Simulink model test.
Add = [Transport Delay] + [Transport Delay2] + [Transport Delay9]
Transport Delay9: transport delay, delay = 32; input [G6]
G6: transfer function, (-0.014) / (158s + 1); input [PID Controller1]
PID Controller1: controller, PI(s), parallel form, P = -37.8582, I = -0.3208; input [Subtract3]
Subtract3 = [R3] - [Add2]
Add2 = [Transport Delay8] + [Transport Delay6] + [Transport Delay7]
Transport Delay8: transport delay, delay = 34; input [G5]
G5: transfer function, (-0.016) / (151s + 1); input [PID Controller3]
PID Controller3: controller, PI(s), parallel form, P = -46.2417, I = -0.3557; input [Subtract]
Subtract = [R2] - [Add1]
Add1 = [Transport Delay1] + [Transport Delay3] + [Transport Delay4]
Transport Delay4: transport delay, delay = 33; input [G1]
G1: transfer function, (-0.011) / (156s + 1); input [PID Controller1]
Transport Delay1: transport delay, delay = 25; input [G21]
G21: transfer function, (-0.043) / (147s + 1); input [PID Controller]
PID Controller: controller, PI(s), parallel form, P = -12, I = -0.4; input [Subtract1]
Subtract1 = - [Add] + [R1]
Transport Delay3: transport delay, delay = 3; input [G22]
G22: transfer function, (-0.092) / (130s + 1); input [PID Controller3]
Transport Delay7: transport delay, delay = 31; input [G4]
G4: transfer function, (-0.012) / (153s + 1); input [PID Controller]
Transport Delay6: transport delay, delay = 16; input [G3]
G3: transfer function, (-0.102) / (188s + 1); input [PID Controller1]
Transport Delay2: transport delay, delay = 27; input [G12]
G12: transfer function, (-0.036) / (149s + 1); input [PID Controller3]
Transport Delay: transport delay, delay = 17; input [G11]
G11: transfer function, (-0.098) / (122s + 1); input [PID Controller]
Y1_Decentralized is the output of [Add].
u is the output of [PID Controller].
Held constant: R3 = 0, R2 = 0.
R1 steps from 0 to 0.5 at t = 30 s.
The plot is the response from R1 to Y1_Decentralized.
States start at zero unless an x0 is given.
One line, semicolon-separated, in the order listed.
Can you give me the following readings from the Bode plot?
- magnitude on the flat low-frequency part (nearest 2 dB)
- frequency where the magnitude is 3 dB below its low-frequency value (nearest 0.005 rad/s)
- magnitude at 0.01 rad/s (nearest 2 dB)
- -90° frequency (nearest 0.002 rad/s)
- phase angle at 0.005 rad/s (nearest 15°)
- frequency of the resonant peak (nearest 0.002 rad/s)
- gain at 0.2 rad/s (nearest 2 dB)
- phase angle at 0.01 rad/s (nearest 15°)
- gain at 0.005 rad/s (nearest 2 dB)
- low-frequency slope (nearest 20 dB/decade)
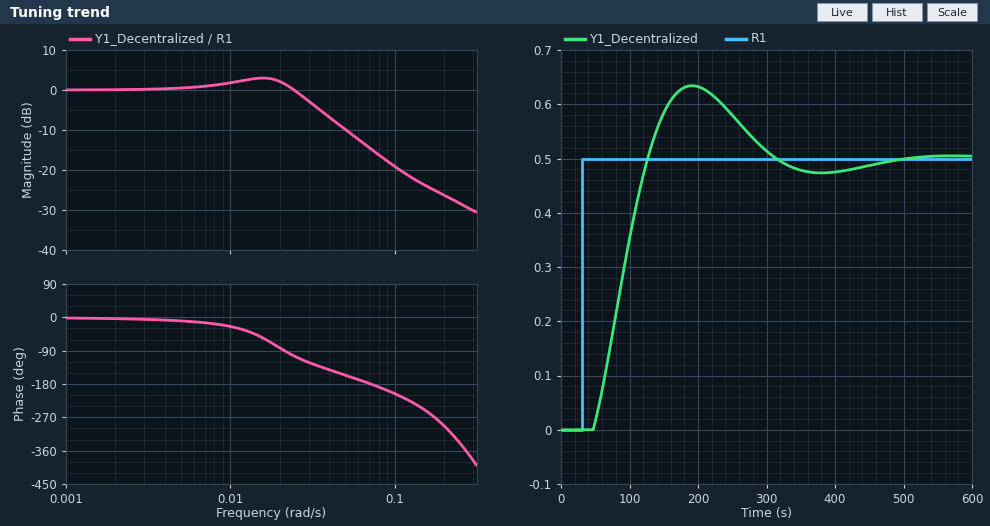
0 dB; 0.030 rad/s; 2 dB; 0.022 rad/s; -15°; 0.016 rad/s; -26 dB; -30°; 0 dB; 0 dB/decade
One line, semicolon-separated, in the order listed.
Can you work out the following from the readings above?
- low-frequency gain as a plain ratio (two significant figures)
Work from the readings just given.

1.0
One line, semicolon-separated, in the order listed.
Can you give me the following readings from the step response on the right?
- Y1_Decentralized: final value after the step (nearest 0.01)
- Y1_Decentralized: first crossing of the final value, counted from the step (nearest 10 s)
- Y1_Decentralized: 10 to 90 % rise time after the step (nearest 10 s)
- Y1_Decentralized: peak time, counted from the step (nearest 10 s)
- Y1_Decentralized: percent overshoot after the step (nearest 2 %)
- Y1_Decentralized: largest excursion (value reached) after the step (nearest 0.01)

0.50; 100 s; 60 s; 160 s; 26 %; 0.63
